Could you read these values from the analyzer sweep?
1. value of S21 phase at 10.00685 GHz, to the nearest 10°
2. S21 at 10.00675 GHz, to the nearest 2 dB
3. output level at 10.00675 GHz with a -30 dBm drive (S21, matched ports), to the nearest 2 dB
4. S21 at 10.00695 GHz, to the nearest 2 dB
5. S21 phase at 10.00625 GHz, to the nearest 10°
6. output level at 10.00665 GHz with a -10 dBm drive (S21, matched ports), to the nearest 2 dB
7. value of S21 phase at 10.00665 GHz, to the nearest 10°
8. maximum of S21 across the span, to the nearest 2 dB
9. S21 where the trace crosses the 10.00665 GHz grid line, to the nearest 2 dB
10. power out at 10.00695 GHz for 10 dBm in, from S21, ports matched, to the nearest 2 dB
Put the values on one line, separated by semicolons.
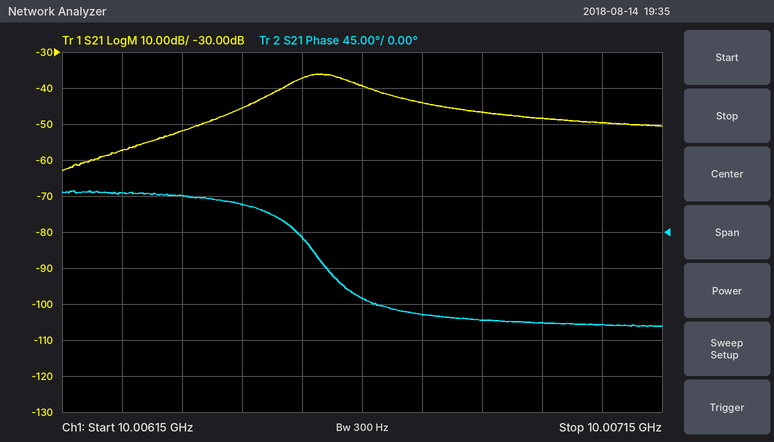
-110°; -44 dB; -74 dBm; -48 dB; 50°; -50 dBm; -80°; -36 dB; -40 dB; -38 dBm
